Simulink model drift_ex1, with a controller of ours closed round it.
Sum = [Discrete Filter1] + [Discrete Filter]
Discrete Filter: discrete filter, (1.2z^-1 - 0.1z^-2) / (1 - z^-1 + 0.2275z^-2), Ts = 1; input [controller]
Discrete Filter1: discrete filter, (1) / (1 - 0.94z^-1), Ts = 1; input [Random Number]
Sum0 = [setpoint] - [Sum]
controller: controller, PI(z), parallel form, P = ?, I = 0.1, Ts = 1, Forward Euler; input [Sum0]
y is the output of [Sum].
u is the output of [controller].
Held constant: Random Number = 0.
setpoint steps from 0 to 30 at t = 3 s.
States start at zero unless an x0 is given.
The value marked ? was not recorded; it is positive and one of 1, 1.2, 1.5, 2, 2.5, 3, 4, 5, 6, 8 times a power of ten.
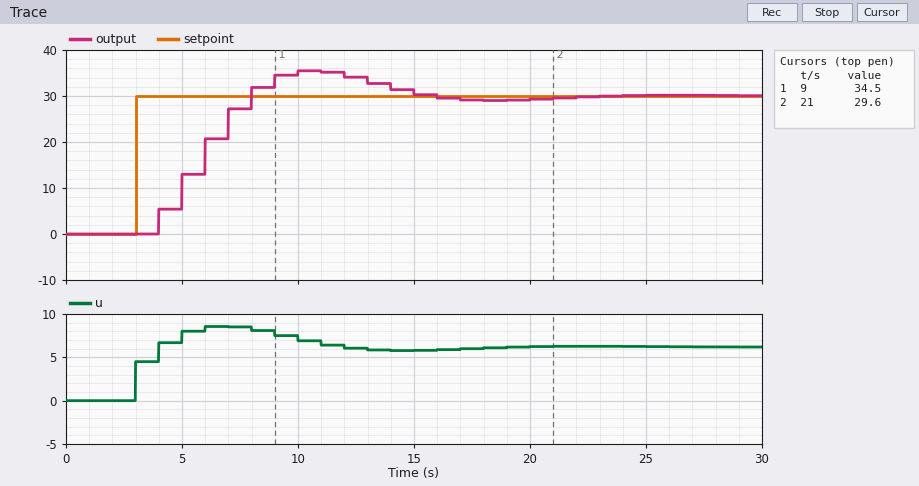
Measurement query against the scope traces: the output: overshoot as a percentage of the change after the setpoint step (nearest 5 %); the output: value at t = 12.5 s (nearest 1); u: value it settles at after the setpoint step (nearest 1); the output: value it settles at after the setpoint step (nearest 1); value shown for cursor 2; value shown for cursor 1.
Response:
20 %
34
6
30
29.6
34.5
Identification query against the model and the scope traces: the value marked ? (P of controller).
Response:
0.15
